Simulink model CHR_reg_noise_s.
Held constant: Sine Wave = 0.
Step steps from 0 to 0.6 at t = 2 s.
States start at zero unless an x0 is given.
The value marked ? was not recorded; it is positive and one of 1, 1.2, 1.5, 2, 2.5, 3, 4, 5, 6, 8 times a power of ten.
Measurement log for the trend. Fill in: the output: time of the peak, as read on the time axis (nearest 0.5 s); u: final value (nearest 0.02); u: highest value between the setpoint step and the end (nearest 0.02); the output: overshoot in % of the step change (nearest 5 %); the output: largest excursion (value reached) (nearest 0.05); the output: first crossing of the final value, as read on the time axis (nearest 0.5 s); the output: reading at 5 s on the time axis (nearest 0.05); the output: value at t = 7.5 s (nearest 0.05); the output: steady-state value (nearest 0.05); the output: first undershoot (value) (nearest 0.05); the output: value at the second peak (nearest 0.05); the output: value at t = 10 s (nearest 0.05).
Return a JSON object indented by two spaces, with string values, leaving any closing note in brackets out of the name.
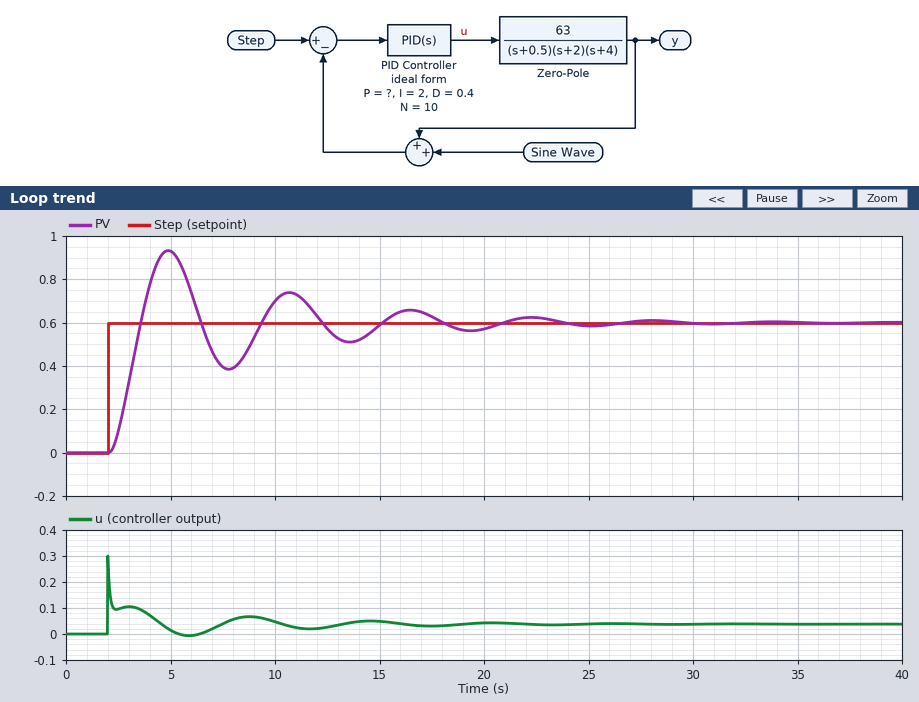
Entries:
{
  "the output: time of the peak, as read on the time axis": "5.0 s",
  "u: final value": "0.04",
  "u: highest value between the setpoint step and the end": "0.30",
  "the output: overshoot in % of the step change": "55 %",
  "the output: largest excursion (value reached)": "0.95",
  "the output: first crossing of the final value, as read on the time axis": "3.5 s",
  "the output: reading at 5 s on the time axis": "0.95",
  "the output: value at t = 7.5 s": "0.40",
  "the output: steady-state value": "0.60",
  "the output: first undershoot (value)": "0.40",
  "the output: value at the second peak": "0.75",
  "the output: value at t = 10 s": "0.70"
}
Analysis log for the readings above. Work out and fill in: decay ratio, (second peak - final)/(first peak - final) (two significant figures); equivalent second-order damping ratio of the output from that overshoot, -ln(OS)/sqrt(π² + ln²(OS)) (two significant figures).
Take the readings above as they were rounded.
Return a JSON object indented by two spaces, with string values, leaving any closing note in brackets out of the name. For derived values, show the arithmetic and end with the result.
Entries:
{
  "decay ratio, (second peak - final)/(first peak - final)": "(0.75 - 0.6) / (0.95 - 0.6) = 0.43",
  "equivalent second-order damping ratio of the output from that overshoot, -ln(OS)/sqrt(π² + ln²(OS))": "ln(0.55) = -0.598; 0.598 / sqrt(9.870 + 0.357) = 0.19"
}
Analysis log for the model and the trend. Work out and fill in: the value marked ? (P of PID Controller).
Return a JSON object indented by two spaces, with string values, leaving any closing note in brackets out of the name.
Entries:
{
  "the value marked ?": "0.1"
}
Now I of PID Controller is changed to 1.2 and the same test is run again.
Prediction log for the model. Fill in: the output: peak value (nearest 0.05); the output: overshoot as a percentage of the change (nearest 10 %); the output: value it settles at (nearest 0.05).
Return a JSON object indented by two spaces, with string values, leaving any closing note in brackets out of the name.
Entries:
{
  "the output: peak value": "0.80",
  "the output: overshoot as a percentage of the change": "30 %",
  "the output: value it settles at": "0.60"
}
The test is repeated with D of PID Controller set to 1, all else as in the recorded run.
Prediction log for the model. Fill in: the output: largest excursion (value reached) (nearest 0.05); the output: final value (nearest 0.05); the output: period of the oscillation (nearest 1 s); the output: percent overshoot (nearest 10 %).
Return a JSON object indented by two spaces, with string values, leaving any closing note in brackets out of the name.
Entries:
{
  "the output: largest excursion (value reached)": "0.80",
  "the output: final value": "0.60",
  "the output: period of the oscillation": "7 s",
  "the output: percent overshoot": "30 %"
}
